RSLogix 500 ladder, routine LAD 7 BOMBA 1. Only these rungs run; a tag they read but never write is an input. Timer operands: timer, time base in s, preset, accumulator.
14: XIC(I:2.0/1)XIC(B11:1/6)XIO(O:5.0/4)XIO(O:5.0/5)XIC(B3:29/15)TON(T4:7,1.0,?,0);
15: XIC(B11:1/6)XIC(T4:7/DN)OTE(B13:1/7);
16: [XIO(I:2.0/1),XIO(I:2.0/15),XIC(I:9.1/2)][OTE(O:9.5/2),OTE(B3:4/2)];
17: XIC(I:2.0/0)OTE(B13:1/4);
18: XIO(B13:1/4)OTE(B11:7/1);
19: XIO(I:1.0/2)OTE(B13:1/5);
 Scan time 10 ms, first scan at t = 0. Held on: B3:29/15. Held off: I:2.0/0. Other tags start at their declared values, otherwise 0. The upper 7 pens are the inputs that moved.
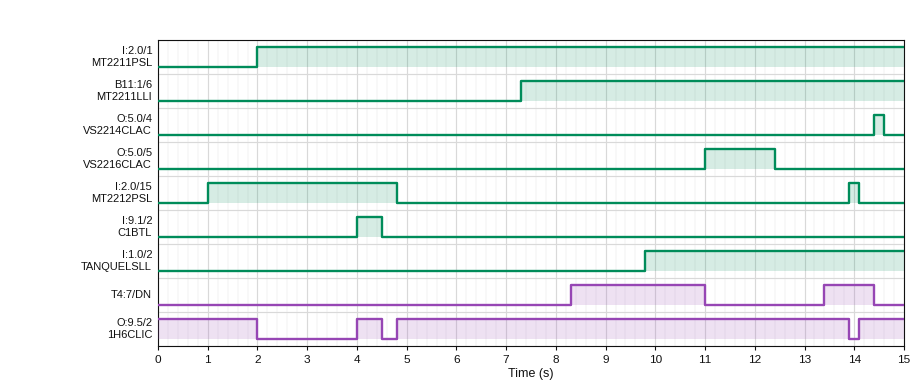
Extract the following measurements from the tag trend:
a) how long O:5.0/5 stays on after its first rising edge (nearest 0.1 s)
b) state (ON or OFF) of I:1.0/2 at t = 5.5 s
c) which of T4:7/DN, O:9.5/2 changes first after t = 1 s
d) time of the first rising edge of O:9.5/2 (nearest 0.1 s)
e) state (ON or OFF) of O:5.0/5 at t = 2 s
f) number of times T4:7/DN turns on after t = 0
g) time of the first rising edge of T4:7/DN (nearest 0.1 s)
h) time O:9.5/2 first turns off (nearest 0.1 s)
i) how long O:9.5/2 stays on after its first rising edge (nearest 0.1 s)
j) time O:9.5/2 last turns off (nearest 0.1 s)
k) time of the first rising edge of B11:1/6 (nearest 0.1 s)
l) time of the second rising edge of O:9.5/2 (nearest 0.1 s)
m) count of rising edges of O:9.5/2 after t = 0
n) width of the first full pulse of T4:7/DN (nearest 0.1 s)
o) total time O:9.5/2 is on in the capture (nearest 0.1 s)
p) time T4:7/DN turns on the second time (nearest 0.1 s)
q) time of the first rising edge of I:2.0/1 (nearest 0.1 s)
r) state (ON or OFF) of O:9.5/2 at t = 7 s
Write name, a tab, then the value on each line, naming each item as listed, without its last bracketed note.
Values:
how long O:5.0/5 stays on after its first rising edge	1.4 s
state (ON or OFF) of I:1.0/2 at t = 5.5 s	OFF
which of T4:7/DN, O:9.5/2 changes first after t = 1 s	O:9.5/2
time of the first rising edge of O:9.5/2	4.0 s
state (ON or OFF) of O:5.0/5 at t = 2 s	OFF
number of times T4:7/DN turns on after t = 0	2
time of the first rising edge of T4:7/DN	8.3 s
time O:9.5/2 first turns off	2.0 s
how long O:9.5/2 stays on after its first rising edge	0.5 s
time O:9.5/2 last turns off	13.9 s
time of the first rising edge of B11:1/6	7.3 s
time of the second rising edge of O:9.5/2	4.8 s
count of rising edges of O:9.5/2 after t = 0	3
width of the first full pulse of T4:7/DN	2.7 s
total time O:9.5/2 is on in the capture	12.5 s
time T4:7/DN turns on the second time	13.4 s
time of the first rising edge of I:2.0/1	2.0 s
state (ON or OFF) of O:9.5/2 at t = 7 s	ON
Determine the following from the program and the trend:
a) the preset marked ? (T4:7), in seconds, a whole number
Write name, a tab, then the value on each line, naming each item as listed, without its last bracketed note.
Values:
the preset marked ? (T4:7), in seconds, a whole number	1 s
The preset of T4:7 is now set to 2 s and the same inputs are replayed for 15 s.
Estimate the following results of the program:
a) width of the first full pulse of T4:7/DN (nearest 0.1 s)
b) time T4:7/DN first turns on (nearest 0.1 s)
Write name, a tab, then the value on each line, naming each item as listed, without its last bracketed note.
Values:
width of the first full pulse of T4:7/DN	1.7 s
time T4:7/DN first turns on	9.3 s
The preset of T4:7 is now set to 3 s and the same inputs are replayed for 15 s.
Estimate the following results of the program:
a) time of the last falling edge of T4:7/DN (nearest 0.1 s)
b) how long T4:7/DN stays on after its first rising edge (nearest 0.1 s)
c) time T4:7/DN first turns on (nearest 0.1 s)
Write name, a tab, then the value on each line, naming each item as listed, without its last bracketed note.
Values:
time of the last falling edge of T4:7/DN	11.0 s
how long T4:7/DN stays on after its first rising edge	0.7 s
time T4:7/DN first turns on	10.3 s
